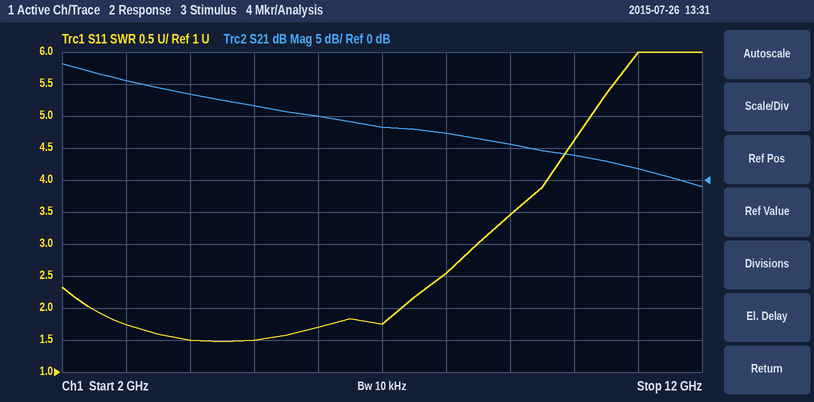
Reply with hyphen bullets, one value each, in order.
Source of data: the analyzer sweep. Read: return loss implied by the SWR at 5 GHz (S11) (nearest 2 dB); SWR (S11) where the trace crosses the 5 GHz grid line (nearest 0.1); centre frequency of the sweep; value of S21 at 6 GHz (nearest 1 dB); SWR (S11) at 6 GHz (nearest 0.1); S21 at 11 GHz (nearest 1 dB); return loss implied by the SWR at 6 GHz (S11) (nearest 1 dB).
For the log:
- 14 dB
- 1.5
- 7 GHz
- 10 dB
- 1.7
- 2 dB
- 12 dB
